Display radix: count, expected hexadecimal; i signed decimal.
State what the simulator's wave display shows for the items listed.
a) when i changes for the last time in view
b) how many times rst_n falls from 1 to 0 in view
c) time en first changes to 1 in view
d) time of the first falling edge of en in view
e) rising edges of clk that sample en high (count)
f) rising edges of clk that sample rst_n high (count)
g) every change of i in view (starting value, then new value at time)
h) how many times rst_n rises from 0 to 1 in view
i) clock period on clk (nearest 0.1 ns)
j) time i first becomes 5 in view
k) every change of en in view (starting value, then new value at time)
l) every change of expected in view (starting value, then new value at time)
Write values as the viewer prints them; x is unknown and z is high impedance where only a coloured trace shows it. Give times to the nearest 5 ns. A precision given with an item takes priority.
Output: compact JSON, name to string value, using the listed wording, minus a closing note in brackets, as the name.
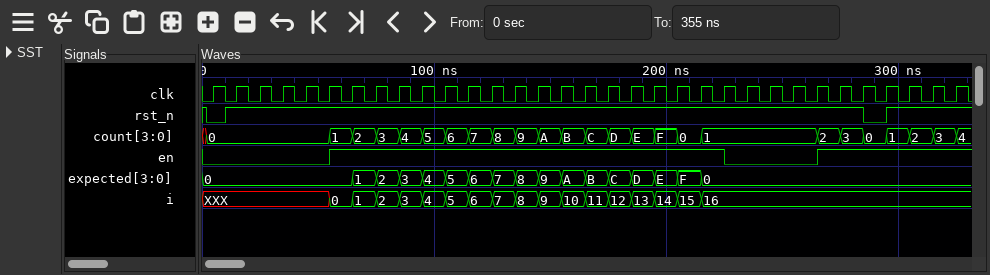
{"when i changes for the last time in view": "215 ns", "how many times rst_n falls from 1 to 0 in view": "2", "time en first changes to 1 in view": "55 ns", "time of the first falling edge of en in view": "225 ns", "rising edges of clk that sample en high": "23", "rising edges of clk that sample rst_n high": "31", "every change of i in view": "XXX, 0 at 55 ns, 1 at 65 ns, 2 at 75 ns, 3 at 85 ns, 4 at 95 ns, 5 at 105 ns, 6 at 115 ns, 7 at 125 ns, 8 at 135 ns, 9 at 145 ns, 10 at 155 ns, 11 at 165 ns, 12 at 175 ns, 13 at 185 ns, 14 at 195 ns, 15 at 205 ns, 16 at 215 ns", "how many times rst_n rises from 0 to 1 in view": "2", "clock period on clk": "10 ns", "time i first becomes 5 in view": "105 ns", "every change of en in view": "0, 1 at 55 ns, 0 at 225 ns, 1 at 265 ns", "every change of expected in view": "0, 1 at 65 ns, 2 at 75 ns, 3 at 85 ns, 4 at 95 ns, 5 at 105 ns, 6 at 115 ns, 7 at 125 ns, 8 at 135 ns, 9 at 145 ns, A at 155 ns, B at 165 ns, C at 175 ns, D at 185 ns, E at 195 ns, F at 205 ns, 0 at 215 ns"}
